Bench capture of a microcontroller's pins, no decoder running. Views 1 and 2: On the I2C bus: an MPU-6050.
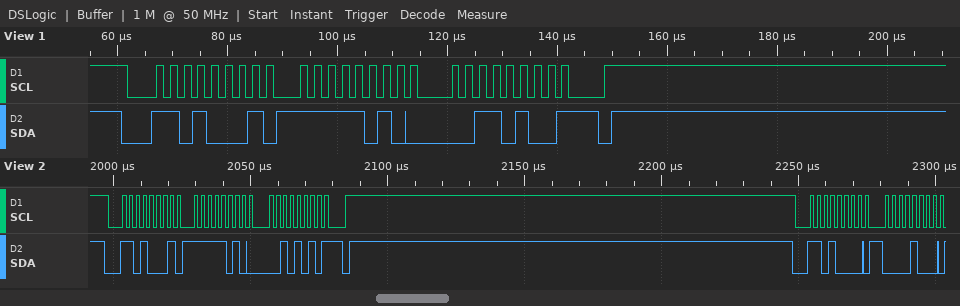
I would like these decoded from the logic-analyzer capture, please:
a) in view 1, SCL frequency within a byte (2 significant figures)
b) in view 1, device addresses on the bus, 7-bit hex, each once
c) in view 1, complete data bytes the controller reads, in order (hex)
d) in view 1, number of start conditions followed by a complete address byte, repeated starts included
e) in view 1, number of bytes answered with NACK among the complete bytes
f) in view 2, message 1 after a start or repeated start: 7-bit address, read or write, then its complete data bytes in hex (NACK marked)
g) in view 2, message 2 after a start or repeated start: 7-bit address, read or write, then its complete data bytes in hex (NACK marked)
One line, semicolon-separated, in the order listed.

400 kHz; 0x68; FA 34; 1; 1; 0x68 read: FA 2A NACK; 0x68 write: 08
